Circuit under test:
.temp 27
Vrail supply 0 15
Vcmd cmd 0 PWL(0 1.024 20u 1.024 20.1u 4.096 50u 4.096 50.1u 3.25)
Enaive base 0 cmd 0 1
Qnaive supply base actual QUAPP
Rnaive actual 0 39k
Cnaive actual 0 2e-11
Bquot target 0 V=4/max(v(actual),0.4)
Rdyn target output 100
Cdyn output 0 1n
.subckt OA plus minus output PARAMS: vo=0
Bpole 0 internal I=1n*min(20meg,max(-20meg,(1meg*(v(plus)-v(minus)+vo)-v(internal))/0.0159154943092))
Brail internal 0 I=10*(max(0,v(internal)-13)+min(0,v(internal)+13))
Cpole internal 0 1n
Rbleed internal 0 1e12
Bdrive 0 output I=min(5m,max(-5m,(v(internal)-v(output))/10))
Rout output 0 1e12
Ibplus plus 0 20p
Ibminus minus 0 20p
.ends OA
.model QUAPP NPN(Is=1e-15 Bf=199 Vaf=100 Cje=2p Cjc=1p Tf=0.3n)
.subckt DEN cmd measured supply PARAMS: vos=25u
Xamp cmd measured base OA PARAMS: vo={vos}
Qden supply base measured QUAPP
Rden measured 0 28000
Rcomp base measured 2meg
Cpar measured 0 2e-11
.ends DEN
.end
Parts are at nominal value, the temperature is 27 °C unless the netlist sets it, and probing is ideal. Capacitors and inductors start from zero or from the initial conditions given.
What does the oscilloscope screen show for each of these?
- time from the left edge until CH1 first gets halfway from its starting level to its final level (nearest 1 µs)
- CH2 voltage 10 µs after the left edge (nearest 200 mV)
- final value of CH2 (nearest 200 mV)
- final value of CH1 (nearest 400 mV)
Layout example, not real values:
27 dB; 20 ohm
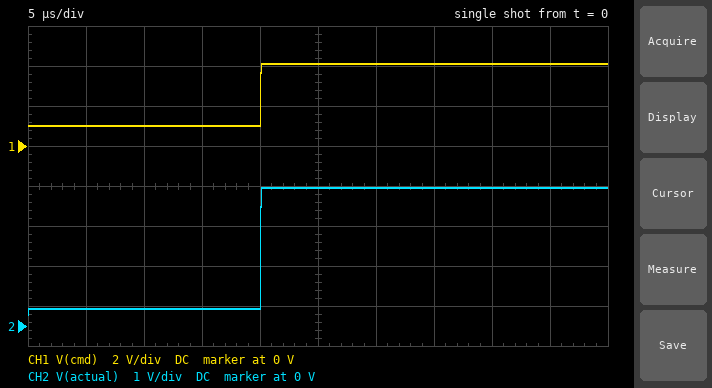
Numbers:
20 µs; 400 mV; 3.4 V; 4.0 V
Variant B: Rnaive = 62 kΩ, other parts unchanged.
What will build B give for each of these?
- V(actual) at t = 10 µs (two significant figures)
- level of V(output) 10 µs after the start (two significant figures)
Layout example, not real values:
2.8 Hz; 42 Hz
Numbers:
440 mV; 9.1 V
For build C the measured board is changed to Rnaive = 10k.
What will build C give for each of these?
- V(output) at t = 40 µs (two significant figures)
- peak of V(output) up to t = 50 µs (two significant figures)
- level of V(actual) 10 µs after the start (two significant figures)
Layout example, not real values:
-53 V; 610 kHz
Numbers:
1.2 V; 10 V; 400 mV
